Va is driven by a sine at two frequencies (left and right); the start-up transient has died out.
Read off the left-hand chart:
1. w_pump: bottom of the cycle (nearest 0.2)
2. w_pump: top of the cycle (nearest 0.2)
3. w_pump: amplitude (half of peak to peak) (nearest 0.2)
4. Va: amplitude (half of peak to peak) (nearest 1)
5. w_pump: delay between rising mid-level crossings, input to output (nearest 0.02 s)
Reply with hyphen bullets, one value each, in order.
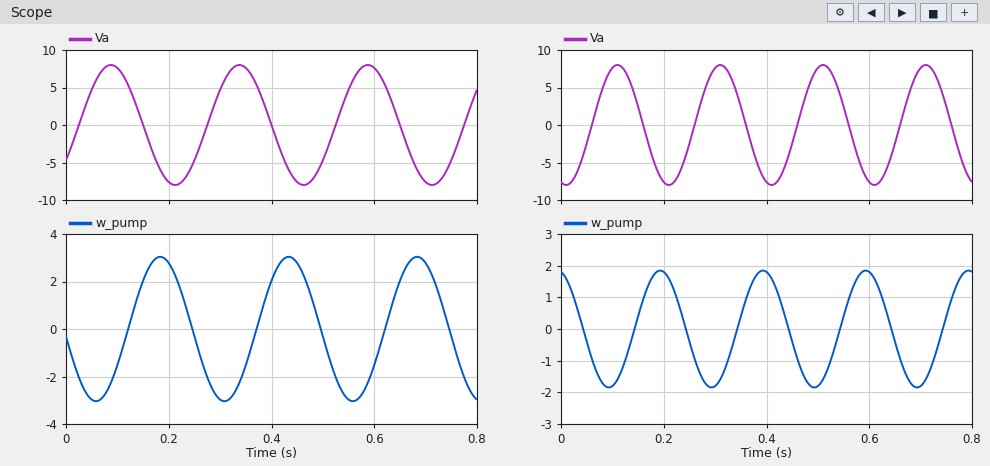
- -3.0
- 3.0
- 3.0
- 8
- 0.10 s
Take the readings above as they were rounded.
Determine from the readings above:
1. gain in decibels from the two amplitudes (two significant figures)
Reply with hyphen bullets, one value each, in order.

- -8.5 dB
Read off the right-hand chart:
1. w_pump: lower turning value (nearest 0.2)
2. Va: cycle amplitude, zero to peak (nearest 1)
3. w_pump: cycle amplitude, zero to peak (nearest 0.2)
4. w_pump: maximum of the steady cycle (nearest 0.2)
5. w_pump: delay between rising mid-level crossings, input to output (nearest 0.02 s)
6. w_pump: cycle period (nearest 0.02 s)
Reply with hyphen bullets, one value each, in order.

- -1.8
- 8
- 1.8
- 1.8
- 0.08 s
- 0.20 s
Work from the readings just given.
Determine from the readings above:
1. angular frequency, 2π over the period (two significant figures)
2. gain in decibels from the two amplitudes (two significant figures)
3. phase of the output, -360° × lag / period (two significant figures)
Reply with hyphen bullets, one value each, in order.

- 31 rad/s
- -13 dB
- -140°
